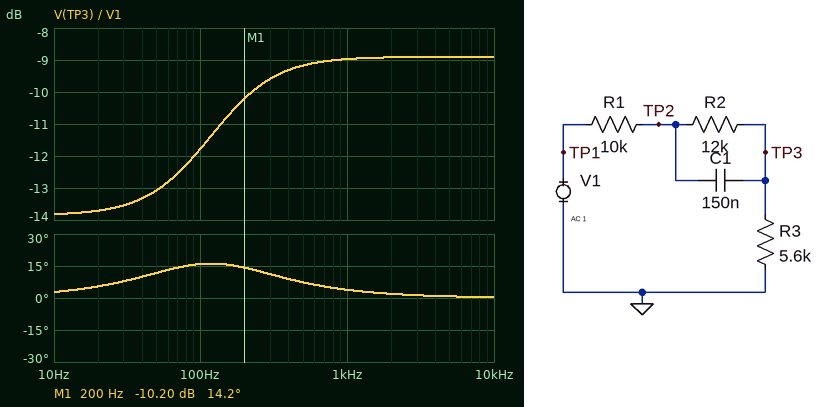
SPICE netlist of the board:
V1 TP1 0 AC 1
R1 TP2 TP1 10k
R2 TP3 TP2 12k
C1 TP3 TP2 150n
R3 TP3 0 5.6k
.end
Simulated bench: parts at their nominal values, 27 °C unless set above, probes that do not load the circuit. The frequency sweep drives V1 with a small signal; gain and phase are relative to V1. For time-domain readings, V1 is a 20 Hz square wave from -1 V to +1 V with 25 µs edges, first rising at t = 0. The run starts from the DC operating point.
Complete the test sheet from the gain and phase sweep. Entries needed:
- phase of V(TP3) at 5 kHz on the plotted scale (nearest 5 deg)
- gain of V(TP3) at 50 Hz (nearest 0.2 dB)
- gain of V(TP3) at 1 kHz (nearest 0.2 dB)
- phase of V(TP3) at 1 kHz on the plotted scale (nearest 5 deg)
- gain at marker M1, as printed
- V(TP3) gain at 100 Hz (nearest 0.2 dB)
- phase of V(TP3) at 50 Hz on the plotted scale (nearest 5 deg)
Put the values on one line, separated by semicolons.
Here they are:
0 deg; -13.0 dB; -9.0 dB; 5 deg; -10.20 dB; -11.8 dB; 10 deg
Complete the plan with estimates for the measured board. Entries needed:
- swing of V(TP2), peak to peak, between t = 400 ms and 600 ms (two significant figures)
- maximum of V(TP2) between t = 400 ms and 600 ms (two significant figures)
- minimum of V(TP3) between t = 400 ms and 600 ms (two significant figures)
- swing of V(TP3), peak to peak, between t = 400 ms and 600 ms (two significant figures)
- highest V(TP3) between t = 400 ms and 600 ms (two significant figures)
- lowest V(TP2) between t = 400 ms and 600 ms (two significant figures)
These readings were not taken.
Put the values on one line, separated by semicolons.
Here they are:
1.3 V; 640 mV; -510 mV; 1.0 V; 510 mV; -640 mV
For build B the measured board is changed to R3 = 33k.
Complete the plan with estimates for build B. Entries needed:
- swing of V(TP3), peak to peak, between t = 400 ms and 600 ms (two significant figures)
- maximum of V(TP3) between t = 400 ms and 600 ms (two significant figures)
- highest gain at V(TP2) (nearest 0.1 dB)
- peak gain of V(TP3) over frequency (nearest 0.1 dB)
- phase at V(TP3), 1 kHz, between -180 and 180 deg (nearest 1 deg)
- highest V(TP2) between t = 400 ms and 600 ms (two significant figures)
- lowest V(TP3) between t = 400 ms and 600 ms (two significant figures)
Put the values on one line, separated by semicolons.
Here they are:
1.9 V; 930 mV; -1.7 dB; -2.3 dB; 1 deg; 820 mV; -930 mV
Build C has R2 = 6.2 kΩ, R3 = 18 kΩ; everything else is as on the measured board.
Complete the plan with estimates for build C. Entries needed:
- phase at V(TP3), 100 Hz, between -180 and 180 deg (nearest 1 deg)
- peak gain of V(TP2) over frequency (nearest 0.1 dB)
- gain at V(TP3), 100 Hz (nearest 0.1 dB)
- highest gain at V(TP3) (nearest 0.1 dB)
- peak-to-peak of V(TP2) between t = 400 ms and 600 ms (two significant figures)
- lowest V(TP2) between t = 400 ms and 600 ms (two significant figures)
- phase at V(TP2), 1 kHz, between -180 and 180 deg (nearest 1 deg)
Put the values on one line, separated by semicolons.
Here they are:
5 deg; -3.0 dB; -5.2 dB; -3.8 dB; 1.4 V; -710 mV; -1 deg
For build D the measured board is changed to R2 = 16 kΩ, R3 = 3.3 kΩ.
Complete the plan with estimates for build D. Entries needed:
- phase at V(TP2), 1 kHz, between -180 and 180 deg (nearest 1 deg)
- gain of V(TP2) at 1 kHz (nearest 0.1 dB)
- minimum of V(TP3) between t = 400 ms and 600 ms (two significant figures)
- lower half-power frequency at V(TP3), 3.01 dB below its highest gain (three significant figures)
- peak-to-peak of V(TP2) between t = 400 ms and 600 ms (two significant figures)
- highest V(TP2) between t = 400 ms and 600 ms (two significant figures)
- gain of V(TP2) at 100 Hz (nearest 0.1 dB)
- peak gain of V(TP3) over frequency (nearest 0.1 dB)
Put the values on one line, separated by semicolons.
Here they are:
-13 deg; -11.6 dB; -380 mV; 112 Hz; 1.3 V; 660 mV; -5.0 dB; -12.1 dB
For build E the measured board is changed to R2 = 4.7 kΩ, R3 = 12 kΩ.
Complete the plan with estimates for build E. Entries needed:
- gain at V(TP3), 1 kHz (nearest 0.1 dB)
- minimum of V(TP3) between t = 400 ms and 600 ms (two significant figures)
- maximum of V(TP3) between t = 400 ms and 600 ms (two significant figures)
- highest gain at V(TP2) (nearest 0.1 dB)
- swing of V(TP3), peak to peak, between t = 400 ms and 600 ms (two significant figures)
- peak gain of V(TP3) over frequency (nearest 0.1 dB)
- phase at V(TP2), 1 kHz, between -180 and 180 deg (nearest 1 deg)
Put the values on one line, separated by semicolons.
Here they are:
-5.4 dB; -640 mV; 640 mV; -4.1 dB; 1.3 V; -5.3 dB; -2 deg
